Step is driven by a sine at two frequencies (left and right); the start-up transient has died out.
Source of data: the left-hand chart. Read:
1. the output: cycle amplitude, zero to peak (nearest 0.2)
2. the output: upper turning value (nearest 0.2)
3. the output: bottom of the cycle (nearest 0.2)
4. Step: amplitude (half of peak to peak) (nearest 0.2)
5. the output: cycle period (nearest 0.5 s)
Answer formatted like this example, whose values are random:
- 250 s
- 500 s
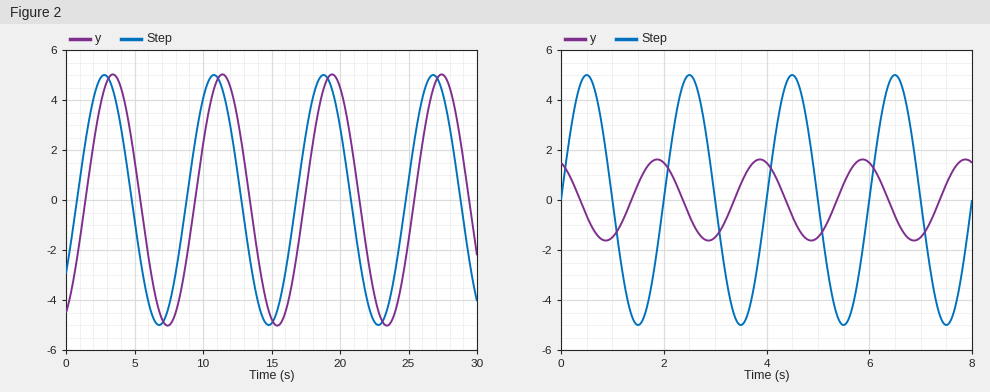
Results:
- 5.0
- 5.0
- -5.0
- 5.0
- 8.0 s
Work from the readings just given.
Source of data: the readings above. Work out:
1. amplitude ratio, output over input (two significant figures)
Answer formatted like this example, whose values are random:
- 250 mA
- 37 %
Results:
- 1.0
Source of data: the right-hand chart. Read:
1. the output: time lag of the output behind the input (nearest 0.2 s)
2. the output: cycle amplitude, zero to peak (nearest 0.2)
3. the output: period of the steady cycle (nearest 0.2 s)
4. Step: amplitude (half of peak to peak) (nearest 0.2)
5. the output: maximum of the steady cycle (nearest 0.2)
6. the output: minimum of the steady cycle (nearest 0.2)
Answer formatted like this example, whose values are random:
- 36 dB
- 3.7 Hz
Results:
- 1.4 s
- 1.6
- 2.0 s
- 5.0
- 1.6
- -1.6
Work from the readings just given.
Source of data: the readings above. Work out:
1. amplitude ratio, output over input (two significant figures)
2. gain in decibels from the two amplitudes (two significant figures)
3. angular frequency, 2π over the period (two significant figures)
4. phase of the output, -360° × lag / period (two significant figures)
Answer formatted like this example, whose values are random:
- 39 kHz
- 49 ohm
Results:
- 0.32
- -9.9 dB
- 3.1 rad/s
- -250°
